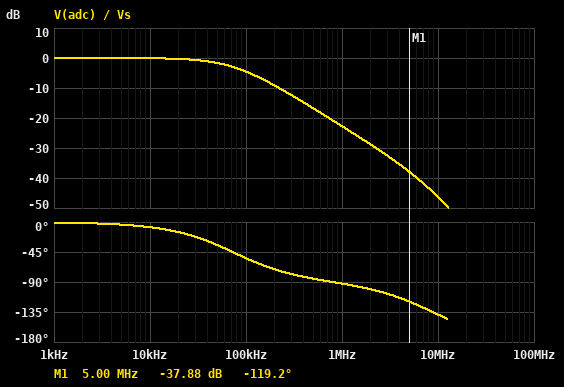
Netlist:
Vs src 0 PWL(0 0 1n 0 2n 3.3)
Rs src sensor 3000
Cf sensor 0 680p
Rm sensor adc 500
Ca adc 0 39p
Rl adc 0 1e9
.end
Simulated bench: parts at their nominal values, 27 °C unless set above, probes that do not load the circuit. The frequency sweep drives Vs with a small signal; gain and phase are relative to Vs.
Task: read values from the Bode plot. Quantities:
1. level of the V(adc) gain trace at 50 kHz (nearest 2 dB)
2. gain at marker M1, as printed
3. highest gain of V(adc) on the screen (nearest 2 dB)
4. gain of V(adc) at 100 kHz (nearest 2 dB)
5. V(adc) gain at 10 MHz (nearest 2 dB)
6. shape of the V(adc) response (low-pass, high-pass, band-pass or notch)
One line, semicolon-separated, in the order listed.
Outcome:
-2 dB; -37.88 dB; 0 dB; -4 dB; -46 dB; low-pass
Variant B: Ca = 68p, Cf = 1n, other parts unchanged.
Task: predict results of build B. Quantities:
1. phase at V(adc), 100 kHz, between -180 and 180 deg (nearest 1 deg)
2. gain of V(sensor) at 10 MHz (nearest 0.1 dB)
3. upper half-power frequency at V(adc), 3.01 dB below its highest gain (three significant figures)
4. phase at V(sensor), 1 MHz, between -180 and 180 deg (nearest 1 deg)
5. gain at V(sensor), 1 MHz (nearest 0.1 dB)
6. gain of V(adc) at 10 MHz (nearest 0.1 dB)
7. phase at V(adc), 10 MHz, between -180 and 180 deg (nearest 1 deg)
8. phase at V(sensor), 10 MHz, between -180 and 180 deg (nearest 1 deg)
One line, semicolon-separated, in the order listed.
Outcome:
-65 deg; -45.6 dB; 49.6 kHz; -86 deg; -26.1 dB; -53.1 dB; -153 deg; -88 deg
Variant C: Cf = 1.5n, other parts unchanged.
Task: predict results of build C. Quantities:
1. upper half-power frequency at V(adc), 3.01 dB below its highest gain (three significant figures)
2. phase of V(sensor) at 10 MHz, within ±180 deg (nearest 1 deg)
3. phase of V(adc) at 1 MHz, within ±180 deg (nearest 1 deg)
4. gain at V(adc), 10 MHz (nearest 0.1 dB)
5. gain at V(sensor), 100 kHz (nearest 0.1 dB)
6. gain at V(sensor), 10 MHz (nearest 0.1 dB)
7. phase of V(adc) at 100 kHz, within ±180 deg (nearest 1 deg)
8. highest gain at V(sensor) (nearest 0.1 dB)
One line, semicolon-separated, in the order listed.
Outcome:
34.5 kHz; -89 deg; -95 deg; -53.1 dB; -9.7 dB; -49.1 dB; -72 deg; 0 dB
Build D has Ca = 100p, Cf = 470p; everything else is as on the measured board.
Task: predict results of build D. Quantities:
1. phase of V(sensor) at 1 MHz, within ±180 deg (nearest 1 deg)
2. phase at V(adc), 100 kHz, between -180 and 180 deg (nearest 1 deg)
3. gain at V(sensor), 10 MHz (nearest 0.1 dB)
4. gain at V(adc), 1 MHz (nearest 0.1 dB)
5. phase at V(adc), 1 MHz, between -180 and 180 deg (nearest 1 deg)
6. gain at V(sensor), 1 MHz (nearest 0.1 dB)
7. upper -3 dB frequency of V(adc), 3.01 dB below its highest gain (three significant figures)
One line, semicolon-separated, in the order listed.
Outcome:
-82 deg; -49 deg; -39.1 dB; -21.0 dB; -99 deg; -20.6 dB; 92.5 kHz
